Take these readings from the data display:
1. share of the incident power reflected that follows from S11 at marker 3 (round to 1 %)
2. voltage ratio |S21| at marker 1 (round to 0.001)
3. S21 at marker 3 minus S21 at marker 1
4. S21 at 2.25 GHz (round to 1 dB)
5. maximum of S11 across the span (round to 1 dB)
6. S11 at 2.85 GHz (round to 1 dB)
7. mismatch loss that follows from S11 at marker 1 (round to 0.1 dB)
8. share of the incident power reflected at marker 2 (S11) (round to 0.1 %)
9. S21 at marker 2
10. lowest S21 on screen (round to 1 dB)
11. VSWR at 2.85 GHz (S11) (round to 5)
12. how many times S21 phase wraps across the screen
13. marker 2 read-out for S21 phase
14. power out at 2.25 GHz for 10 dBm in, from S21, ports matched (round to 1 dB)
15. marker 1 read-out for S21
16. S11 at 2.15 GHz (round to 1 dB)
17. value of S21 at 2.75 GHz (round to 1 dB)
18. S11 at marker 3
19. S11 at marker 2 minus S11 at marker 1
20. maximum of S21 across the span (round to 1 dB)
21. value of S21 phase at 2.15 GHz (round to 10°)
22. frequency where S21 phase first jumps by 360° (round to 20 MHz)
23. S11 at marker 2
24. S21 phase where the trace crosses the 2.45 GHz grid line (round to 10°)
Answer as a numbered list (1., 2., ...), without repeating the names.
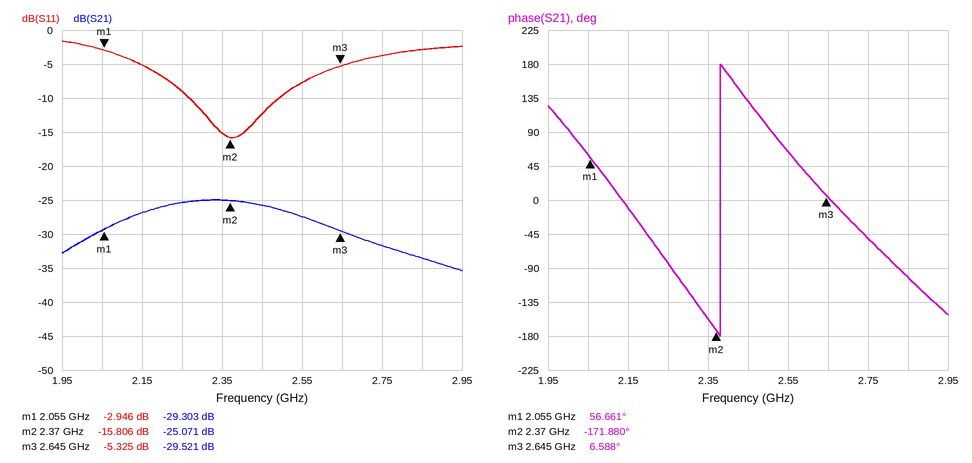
1. 29 %
2. 0.034
3. -0.218 dB
4. -25 dB
5. -2 dB
6. -3 dB
7. 3.1 dB
8. 2.6 %
9. -25.071 dB
10. -35 dB
11. 5
12. 1
13. -171.880°
14. -15 dBm
15. -29.303 dB
16. -5 dB
17. -32 dB
18. -5.325 dB
19. -12.860 dB
20. -25 dB
21. -10°
22. 2.38 GHz
23. -15.806 dB
24. 130°
